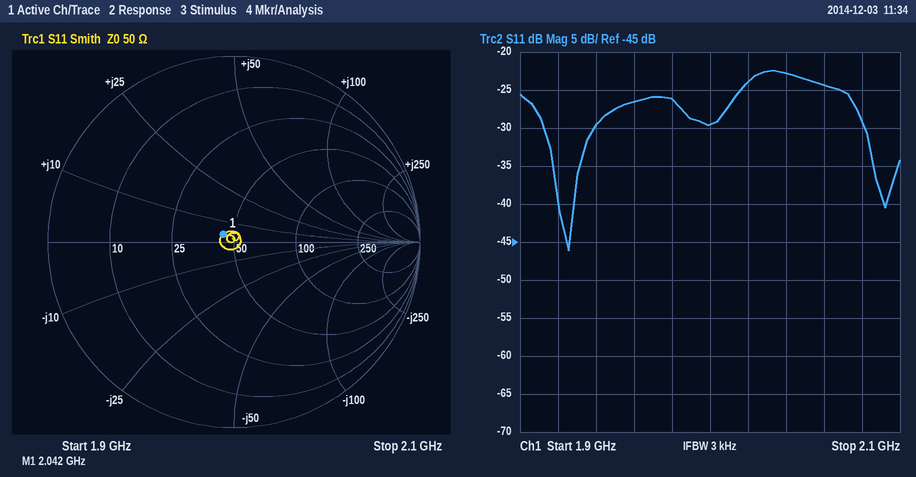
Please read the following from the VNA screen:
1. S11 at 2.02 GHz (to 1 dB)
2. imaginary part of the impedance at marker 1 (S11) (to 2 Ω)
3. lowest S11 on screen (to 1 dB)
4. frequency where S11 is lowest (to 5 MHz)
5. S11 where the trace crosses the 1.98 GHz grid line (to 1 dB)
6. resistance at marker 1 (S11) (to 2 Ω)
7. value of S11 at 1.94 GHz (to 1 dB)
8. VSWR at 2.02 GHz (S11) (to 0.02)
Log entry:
-24 dB
+4 Ω
-46 dB
1.925 GHz
-26 dB
44 Ω
-30 dB
1.14
